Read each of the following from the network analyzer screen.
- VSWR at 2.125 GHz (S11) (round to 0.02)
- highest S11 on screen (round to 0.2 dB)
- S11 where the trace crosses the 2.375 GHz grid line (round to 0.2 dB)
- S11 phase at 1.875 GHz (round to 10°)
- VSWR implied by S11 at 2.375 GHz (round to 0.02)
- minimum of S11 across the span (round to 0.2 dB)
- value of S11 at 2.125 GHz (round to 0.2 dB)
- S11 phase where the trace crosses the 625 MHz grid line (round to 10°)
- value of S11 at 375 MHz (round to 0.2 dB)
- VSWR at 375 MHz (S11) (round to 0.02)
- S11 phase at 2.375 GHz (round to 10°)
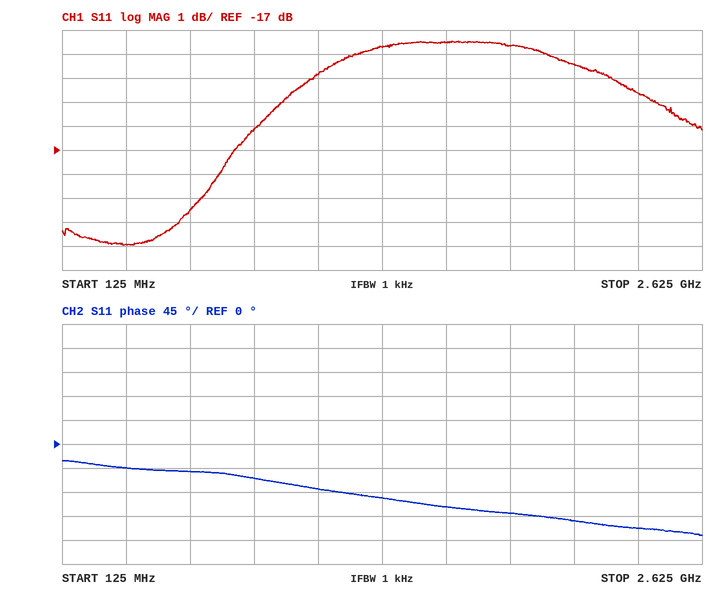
1.54
-12.4 dB
-14.6 dB
-130°
1.46
-21.0 dB
-13.4 dB
-50°
-21.0 dB
1.20
-160°
